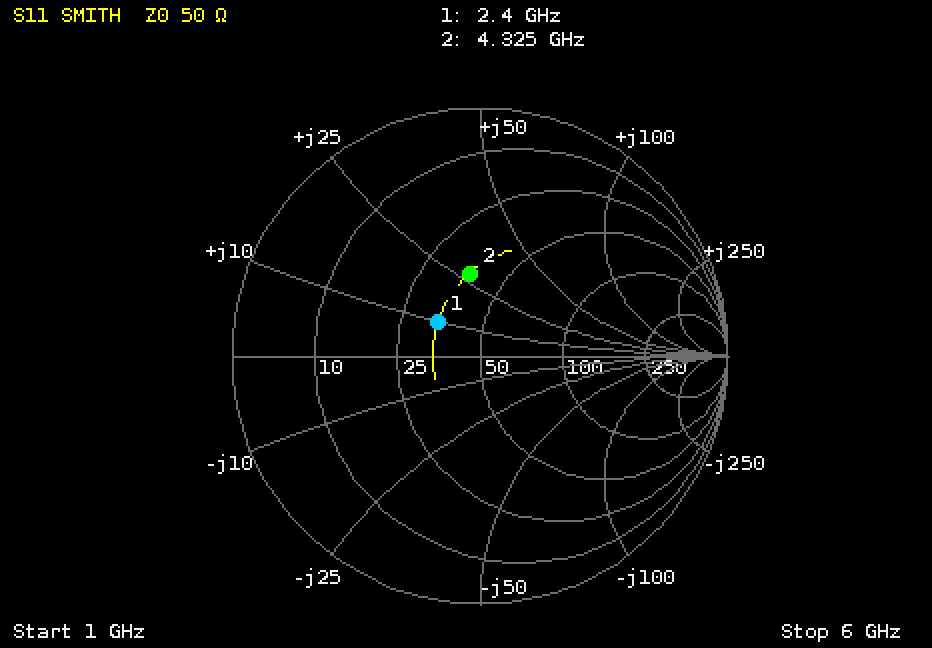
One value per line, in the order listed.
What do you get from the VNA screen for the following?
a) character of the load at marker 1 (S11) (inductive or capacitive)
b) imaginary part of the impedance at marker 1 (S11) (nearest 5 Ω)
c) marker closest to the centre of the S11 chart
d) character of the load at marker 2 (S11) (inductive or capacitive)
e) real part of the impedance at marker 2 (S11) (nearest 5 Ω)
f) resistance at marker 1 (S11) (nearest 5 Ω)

inductive
+10 Ω
marker 1
inductive
35 Ω
35 Ω
